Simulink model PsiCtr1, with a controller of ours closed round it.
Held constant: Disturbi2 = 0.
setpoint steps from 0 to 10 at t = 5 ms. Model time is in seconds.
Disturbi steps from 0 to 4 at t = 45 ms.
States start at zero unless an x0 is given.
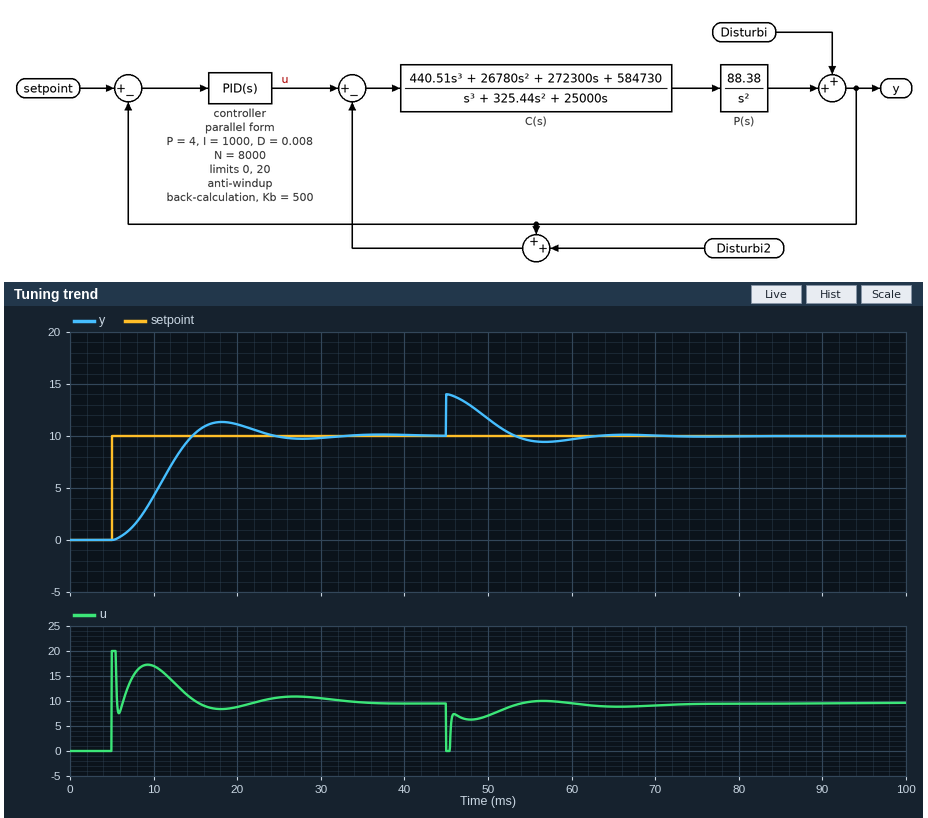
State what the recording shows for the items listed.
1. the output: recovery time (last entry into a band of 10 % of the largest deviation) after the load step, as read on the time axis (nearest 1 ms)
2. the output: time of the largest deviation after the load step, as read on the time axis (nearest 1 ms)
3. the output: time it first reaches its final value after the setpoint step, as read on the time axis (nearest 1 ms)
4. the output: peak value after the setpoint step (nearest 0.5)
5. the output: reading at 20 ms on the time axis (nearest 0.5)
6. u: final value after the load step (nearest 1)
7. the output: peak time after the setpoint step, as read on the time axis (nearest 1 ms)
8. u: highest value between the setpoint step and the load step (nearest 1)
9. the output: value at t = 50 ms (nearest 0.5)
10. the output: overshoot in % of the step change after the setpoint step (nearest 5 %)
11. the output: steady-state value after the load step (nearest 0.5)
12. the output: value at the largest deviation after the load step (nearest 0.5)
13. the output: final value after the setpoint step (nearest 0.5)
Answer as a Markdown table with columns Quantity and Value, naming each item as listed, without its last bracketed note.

| Quantity | Value |
|---|---|
| the output: recovery time (last entry into a band of 10 % of the largest deviation) after the load step, as read on the time axis | 59 ms |
| the output: time of the largest deviation after the load step, as read on the time axis | 45 ms |
| the output: time it first reaches its final value after the setpoint step, as read on the time axis | 15 ms |
| the output: peak value after the setpoint step | 11.5 |
| the output: reading at 20 ms on the time axis | 11.0 |
| u: final value after the load step | 10 |
| the output: peak time after the setpoint step, as read on the time axis | 18 ms |
| u: highest value between the setpoint step and the load step | 20 |
| the output: value at t = 50 ms | 11.5 |
| the output: overshoot in % of the step change after the setpoint step | 15 % |
| the output: steady-state value after the load step | 10.0 |
| the output: value at the largest deviation after the load step | 14.0 |
| the output: final value after the setpoint step | 10.0 |
